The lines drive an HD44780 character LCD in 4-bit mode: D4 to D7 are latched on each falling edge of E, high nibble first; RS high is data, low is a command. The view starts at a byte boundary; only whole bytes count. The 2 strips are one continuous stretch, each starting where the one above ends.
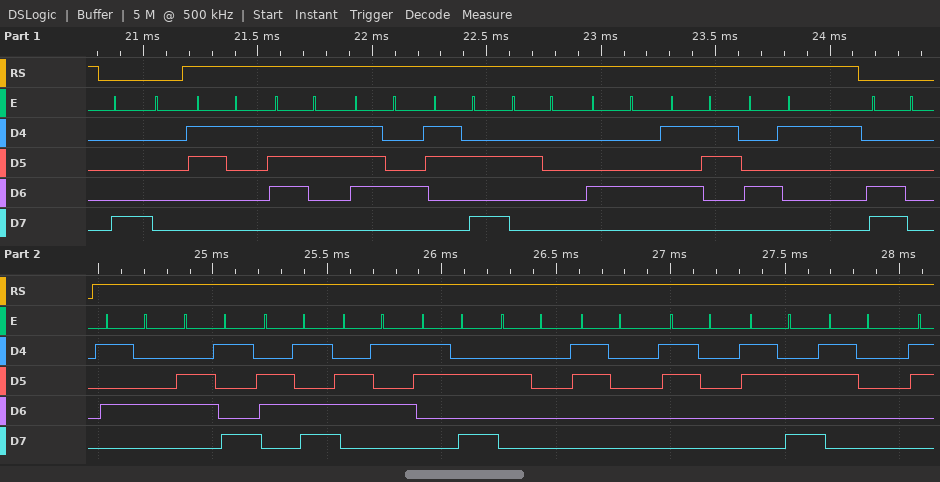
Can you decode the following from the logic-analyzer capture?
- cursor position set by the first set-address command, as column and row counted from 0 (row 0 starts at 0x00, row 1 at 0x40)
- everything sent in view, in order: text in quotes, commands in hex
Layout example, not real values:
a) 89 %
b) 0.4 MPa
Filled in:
a) column 0, row 0
b) 0x80 "1st: DSA" 0xC0 "Time: 00:0"
